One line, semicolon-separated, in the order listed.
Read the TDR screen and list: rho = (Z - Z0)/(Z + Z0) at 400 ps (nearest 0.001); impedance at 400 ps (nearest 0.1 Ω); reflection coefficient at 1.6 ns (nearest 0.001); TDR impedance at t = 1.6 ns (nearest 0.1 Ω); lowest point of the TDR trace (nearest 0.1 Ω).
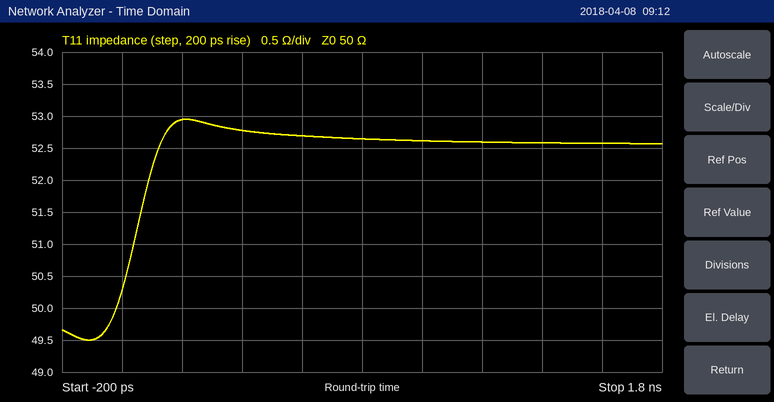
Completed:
+0.027; 52.8 Ω; +0.025; 52.6 Ω; 49.5 Ω
